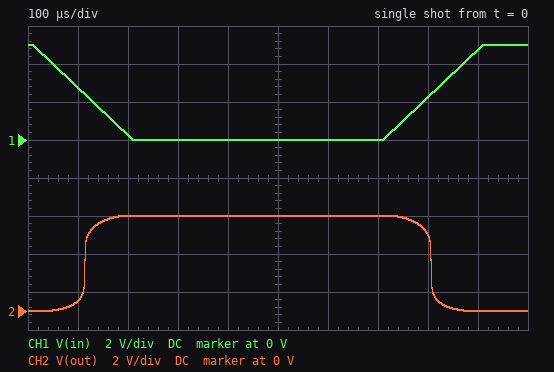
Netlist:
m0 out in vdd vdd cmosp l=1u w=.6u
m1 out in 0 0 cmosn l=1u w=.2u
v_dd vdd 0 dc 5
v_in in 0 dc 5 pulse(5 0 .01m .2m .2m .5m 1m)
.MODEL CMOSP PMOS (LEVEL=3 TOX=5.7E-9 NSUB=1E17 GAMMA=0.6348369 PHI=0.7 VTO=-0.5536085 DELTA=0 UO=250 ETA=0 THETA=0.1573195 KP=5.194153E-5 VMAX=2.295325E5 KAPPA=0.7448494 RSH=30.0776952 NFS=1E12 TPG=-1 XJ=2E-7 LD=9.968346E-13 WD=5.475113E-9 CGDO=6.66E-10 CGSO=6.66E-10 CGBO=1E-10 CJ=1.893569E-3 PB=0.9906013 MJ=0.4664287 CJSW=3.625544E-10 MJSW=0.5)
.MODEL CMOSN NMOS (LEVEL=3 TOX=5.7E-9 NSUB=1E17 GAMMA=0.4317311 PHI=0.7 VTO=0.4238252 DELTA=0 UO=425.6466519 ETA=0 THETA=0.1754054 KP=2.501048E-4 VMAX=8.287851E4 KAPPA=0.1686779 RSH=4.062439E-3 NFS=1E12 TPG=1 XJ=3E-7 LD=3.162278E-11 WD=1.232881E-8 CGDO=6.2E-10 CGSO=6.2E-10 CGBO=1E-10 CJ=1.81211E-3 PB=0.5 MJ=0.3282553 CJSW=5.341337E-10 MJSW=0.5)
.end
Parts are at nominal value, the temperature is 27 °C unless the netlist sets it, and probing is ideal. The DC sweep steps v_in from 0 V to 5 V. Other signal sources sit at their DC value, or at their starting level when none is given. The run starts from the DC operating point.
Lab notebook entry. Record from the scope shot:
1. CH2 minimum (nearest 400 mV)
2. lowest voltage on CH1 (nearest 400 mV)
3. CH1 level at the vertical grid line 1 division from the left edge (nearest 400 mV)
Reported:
0 V
0 V
2.8 V
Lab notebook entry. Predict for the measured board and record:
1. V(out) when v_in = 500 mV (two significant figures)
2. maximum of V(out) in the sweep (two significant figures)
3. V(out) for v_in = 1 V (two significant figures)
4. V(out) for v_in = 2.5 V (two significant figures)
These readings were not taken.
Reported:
5.0 V
5.0 V
4.9 V
950 mV
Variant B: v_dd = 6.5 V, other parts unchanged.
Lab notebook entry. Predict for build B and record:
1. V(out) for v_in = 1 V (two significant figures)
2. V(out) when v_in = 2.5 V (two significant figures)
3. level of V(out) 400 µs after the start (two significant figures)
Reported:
6.4 V
5.8 V
6.5 V
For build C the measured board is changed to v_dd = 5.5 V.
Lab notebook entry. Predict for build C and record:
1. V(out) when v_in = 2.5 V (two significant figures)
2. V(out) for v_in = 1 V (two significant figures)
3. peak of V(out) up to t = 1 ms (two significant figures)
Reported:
4.4 V
5.4 V
5.5 V
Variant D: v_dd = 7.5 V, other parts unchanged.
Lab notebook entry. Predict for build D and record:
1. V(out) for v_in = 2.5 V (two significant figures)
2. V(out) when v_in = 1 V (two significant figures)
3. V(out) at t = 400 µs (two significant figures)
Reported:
6.9 V
7.4 V
7.5 V
